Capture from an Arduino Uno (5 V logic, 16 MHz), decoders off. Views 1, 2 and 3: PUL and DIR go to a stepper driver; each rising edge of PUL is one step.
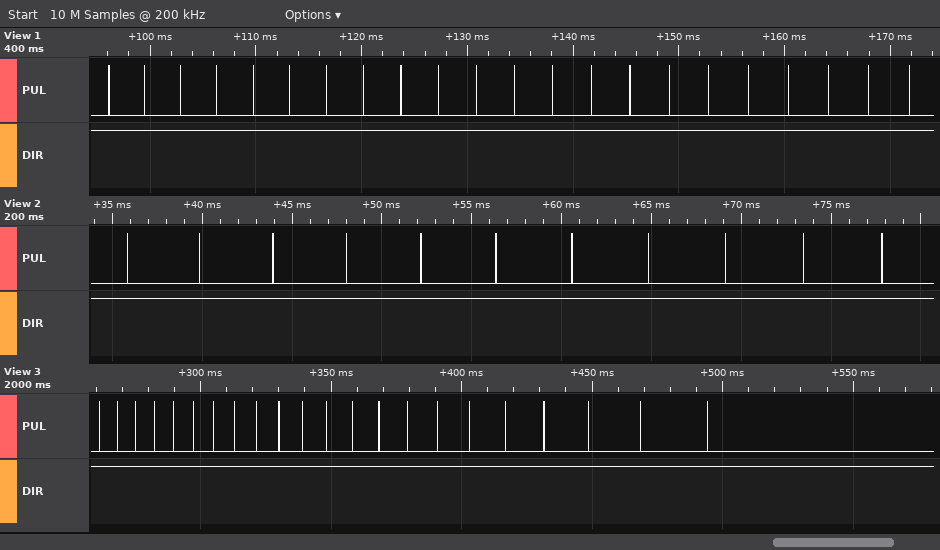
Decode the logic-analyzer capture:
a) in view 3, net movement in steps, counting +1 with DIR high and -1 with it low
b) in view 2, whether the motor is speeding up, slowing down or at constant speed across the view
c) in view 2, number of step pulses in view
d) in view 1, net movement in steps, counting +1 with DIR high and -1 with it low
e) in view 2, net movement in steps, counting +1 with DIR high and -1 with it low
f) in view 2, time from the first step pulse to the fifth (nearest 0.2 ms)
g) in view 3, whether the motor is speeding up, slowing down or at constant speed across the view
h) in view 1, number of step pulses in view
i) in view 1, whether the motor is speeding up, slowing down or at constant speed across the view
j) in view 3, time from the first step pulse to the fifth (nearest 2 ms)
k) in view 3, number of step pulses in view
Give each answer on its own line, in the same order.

+22
slowing down
11
+22
+11
16.4 ms
slowing down
22
slowing down
28 ms
22
